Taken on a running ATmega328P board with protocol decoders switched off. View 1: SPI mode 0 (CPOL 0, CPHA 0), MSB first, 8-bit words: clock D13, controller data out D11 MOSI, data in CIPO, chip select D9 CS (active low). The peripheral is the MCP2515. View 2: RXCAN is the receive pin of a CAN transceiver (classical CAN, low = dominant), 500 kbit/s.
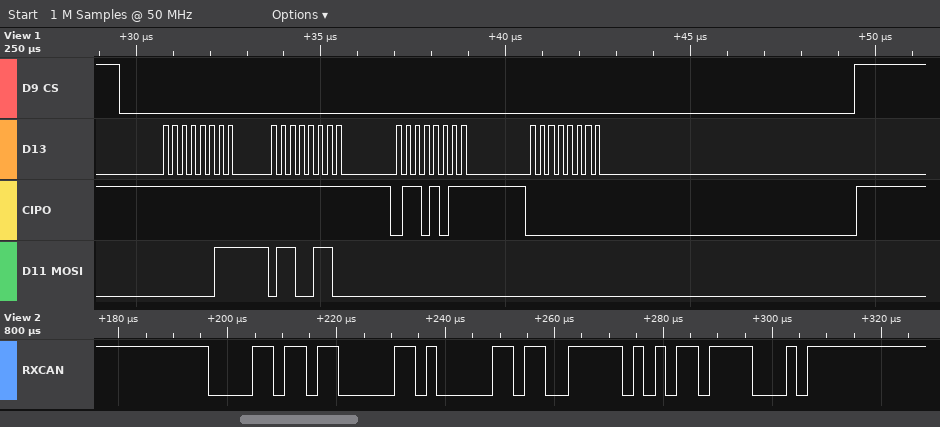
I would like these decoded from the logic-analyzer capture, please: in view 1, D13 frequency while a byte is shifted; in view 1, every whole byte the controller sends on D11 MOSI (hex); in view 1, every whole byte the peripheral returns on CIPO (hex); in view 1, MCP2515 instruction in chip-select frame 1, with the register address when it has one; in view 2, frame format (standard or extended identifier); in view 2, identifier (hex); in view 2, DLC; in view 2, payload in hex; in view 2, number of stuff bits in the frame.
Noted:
4 MHz
03 66 00 00
FF FF 6B 00
READ 0x66
standard
0x0DB
2
82 CF
3
